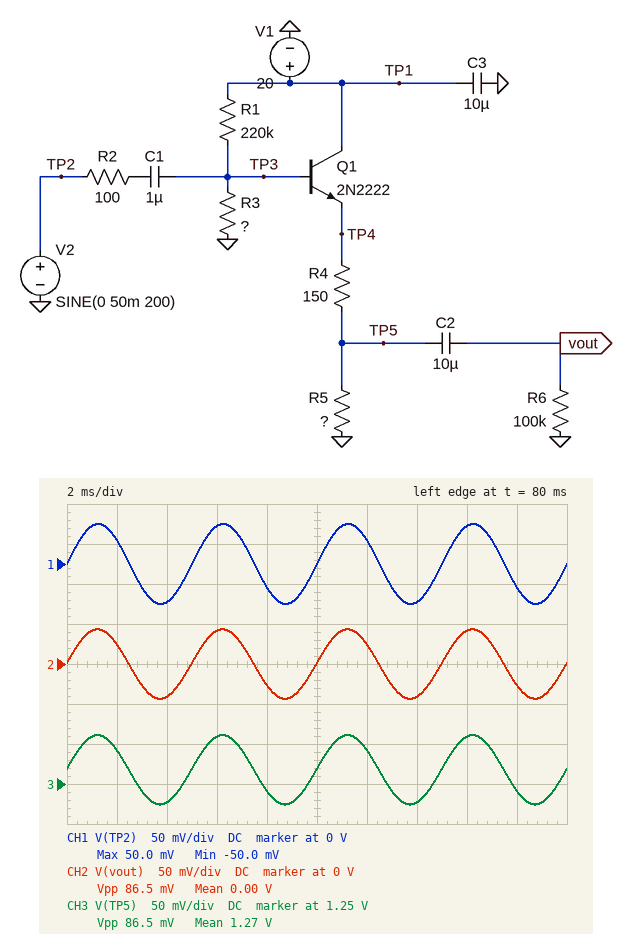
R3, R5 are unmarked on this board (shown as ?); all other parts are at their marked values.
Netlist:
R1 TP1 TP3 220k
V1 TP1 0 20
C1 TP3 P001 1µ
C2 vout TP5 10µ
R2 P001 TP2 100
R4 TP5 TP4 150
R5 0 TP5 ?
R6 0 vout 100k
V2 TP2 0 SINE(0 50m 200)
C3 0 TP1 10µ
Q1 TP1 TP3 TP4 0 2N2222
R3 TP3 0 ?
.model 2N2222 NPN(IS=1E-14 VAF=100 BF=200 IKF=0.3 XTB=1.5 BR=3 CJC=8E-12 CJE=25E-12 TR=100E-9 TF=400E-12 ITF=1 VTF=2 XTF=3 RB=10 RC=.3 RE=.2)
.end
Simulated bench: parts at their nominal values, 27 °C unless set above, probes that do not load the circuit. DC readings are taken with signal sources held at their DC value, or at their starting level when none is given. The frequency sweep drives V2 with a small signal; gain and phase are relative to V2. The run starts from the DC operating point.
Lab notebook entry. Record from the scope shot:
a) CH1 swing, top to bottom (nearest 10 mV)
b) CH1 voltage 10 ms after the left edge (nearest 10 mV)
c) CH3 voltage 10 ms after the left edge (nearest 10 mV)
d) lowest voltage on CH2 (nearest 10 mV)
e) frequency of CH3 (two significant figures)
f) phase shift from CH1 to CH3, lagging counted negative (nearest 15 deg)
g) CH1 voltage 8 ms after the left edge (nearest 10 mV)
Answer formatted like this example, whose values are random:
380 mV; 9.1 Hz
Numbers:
100 mV; 0 V; 1.27 V; -40 mV; 200 Hz; 0 deg; -30 mV
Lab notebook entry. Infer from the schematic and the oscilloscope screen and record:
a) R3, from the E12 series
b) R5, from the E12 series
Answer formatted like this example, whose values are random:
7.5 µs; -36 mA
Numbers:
27 kΩ; 1.2 kΩ
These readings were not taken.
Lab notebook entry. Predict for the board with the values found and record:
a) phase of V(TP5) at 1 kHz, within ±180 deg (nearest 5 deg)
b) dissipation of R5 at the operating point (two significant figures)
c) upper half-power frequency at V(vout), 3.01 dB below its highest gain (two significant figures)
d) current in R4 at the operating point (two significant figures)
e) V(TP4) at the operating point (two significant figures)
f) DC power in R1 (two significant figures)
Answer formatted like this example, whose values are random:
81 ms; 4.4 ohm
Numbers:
0 deg; 1.3 mW; 490 MHz; 1.1 mA; 1.4 V; 1.5 mW
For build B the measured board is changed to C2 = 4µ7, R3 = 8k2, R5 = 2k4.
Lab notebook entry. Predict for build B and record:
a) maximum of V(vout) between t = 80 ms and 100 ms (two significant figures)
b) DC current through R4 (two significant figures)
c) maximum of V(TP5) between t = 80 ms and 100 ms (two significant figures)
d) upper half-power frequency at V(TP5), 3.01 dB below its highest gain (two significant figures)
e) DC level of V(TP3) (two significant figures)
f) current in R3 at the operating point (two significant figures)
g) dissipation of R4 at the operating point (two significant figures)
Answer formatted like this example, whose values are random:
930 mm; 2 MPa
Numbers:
40 mV; 55 µA; 170 mV; 570 MHz; 720 mV; 87 µA; 460 nW
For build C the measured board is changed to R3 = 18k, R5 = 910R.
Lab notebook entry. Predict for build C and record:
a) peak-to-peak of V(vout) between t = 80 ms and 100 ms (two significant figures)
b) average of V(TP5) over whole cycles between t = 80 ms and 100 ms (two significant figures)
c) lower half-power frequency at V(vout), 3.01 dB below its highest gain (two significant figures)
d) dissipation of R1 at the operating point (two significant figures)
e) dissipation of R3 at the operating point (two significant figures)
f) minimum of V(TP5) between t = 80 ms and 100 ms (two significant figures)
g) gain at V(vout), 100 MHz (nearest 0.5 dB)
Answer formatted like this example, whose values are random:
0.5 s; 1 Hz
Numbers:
82 mV; 700 mV; 10 Hz; 1.6 mW; 120 µW; 660 mV; -2.0 dB
